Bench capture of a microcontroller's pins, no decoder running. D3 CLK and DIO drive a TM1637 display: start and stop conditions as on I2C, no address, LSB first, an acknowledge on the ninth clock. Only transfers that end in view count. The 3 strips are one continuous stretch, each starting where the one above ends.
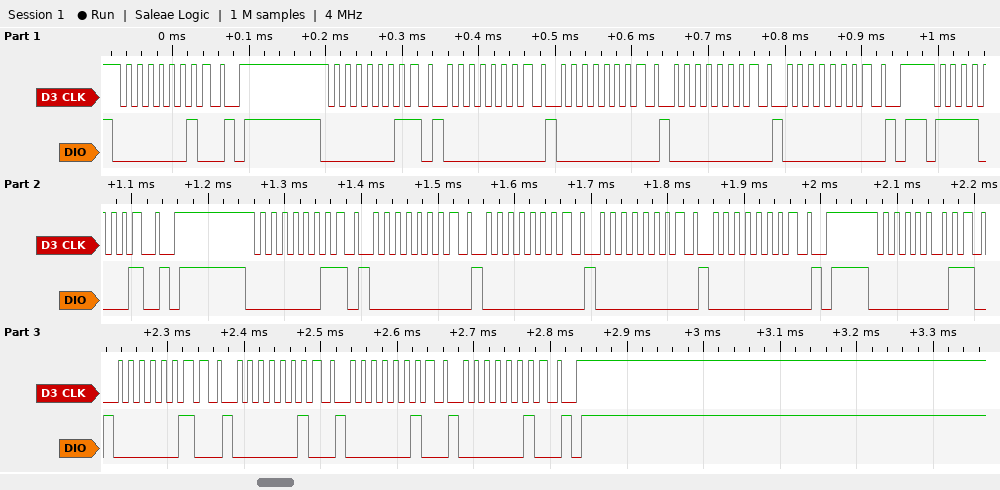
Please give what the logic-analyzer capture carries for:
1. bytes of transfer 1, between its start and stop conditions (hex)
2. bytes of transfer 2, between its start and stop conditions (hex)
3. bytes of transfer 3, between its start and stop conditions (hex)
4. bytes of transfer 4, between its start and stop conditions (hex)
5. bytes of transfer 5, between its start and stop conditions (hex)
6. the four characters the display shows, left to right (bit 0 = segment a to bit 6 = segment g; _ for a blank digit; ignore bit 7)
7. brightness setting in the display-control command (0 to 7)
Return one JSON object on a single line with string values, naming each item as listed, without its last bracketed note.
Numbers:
{"bytes of transfer 1, between its start and stop conditions": "40", "bytes of transfer 2, between its start and stop conditions": "C0 00 00 00 00", "bytes of transfer 3, between its start and stop conditions": "8F", "bytes of transfer 4, between its start and stop conditions": "C0 00 00 00 00", "bytes of transfer 5, between its start and stop conditions": "C0 40 40 40 40", "the four characters the display shows, left to right": "----", "brightness setting in the display-control command": "7"}
